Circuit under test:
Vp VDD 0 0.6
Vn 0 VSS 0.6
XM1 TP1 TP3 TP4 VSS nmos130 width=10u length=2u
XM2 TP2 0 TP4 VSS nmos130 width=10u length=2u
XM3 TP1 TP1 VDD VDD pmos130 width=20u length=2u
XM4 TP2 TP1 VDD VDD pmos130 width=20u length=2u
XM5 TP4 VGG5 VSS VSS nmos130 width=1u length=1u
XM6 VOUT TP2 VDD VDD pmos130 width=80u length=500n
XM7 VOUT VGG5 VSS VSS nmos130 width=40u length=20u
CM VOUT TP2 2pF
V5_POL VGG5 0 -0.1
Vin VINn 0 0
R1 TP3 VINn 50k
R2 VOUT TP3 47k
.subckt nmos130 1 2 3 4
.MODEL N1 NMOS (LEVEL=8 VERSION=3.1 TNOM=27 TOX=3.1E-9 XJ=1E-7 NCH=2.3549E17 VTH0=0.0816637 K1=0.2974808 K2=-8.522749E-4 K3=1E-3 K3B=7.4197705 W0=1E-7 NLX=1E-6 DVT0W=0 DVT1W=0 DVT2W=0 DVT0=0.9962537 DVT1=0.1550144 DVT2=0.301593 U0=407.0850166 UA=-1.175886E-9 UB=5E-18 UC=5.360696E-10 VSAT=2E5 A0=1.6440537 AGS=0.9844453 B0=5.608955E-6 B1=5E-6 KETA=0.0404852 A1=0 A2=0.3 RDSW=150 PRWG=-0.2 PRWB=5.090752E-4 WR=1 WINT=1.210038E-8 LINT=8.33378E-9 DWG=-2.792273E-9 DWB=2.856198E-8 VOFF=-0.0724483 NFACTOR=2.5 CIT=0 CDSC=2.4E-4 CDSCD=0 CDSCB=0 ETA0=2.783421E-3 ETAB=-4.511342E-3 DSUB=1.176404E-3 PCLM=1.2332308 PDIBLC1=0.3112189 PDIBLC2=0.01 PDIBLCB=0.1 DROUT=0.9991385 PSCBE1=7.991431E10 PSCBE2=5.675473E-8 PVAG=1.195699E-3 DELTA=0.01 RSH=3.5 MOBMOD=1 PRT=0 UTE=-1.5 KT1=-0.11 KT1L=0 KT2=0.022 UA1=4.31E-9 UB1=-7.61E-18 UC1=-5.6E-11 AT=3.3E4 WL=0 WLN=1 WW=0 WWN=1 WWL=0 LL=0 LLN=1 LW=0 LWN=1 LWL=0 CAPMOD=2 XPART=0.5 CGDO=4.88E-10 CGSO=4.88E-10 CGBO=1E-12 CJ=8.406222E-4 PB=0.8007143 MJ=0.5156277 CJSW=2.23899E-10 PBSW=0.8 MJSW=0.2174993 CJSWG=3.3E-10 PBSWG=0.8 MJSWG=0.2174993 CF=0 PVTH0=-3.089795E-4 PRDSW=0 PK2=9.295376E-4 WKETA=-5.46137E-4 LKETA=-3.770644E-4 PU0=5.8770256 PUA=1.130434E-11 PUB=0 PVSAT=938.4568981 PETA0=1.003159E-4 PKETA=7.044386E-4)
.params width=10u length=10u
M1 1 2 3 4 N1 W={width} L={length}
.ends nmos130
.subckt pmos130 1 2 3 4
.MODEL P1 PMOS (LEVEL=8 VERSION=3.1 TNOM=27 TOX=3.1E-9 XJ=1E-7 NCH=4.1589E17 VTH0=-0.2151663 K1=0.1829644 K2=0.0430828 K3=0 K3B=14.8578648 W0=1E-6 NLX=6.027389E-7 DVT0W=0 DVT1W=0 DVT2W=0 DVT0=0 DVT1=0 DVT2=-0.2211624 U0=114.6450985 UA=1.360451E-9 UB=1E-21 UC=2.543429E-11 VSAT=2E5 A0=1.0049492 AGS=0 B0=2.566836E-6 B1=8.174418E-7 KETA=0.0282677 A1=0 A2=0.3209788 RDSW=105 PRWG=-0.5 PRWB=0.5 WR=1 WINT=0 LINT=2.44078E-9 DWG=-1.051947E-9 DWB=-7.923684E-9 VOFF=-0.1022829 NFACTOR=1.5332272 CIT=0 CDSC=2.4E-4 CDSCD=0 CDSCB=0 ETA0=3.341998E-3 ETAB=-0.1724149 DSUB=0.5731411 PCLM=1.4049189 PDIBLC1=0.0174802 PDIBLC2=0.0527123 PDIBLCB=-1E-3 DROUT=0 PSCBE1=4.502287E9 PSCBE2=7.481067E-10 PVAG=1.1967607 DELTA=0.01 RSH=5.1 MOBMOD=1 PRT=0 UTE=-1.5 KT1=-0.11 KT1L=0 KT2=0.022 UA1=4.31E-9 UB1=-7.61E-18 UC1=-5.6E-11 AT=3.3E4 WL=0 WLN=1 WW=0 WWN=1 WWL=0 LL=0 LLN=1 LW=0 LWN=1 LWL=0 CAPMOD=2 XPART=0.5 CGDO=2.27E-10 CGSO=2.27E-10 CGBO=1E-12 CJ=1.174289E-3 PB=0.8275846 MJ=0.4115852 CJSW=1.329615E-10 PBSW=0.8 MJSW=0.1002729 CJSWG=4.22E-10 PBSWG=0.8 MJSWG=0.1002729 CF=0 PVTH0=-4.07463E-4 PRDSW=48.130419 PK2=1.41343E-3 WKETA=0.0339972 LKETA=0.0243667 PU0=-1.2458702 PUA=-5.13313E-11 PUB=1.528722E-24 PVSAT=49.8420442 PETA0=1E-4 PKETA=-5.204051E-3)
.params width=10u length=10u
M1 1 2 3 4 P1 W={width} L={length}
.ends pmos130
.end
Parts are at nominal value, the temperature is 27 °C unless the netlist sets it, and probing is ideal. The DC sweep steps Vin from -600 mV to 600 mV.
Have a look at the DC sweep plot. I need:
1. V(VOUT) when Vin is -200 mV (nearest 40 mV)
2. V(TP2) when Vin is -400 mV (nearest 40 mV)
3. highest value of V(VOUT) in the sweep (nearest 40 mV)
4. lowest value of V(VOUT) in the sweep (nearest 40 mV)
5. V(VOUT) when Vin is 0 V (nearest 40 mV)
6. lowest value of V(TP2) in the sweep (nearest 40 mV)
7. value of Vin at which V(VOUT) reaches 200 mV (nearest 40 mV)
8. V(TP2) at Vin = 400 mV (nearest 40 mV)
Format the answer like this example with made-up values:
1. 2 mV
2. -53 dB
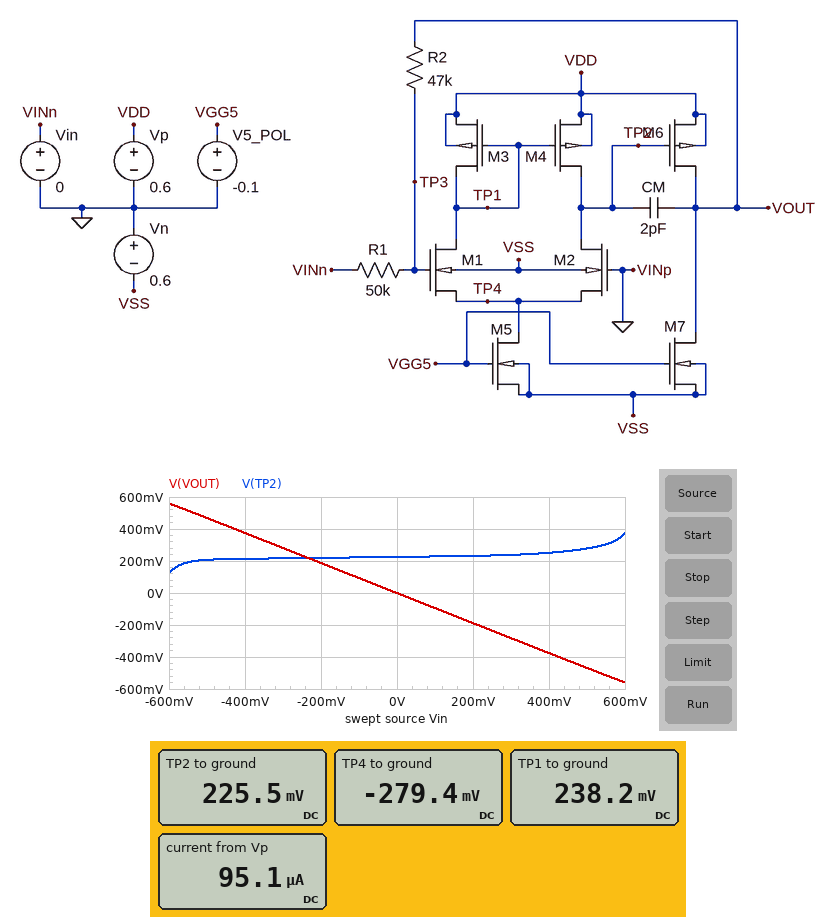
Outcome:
1. 200 mV
2. 200 mV
3. 560 mV
4. -560 mV
5. 0 V
6. 120 mV
7. -200 mV
8. 240 mV
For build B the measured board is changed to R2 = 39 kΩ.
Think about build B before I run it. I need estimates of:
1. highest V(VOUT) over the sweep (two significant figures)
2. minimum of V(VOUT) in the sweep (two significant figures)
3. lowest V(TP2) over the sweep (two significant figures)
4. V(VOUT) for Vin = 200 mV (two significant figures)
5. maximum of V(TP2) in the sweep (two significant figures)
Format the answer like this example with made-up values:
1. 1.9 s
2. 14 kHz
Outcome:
1. 470 mV
2. -470 mV
3. 210 mV
4. -160 mV
5. 280 mV
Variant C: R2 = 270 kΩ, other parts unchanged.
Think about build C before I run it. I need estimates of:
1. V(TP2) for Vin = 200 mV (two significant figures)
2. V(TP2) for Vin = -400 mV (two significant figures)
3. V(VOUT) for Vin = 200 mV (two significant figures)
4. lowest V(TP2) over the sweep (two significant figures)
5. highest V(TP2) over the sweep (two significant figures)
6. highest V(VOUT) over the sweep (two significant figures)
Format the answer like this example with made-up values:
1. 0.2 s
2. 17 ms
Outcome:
1. 570 mV
2. -470 mV
3. -590 mV
4. -570 mV
5. 600 mV
6. 590 mV
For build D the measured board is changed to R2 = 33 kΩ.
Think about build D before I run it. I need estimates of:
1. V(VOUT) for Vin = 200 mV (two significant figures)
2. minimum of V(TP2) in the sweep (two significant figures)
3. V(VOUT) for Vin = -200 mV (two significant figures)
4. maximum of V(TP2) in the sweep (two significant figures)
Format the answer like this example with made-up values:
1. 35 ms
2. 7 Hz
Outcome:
1. -130 mV
2. 210 mV
3. 130 mV
4. 260 mV
